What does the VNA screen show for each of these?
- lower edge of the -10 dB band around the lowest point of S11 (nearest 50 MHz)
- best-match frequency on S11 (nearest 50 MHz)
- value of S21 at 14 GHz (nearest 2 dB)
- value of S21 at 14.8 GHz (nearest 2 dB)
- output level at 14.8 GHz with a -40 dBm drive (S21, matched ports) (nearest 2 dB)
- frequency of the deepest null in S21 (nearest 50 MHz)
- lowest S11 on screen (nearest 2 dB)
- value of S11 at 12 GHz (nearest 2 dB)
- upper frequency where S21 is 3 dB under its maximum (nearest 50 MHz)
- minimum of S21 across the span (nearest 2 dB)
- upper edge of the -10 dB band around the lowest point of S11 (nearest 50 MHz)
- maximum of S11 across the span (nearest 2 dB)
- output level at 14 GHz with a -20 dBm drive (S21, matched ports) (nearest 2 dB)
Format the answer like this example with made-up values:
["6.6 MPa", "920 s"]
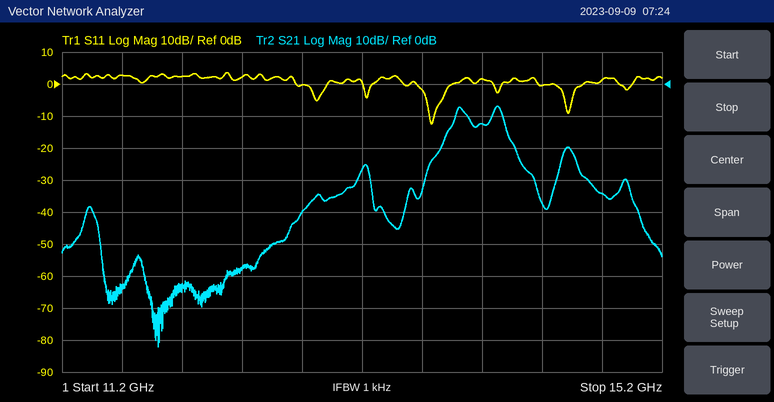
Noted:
["13.65 GHz", "13.65 GHz", "-12 dB", "-34 dB", "-74 dBm", "11.85 GHz", "-12 dB", "2 dB", "14.15 GHz", "-82 dB", "13.70 GHz", "4 dB", "-32 dBm"]
